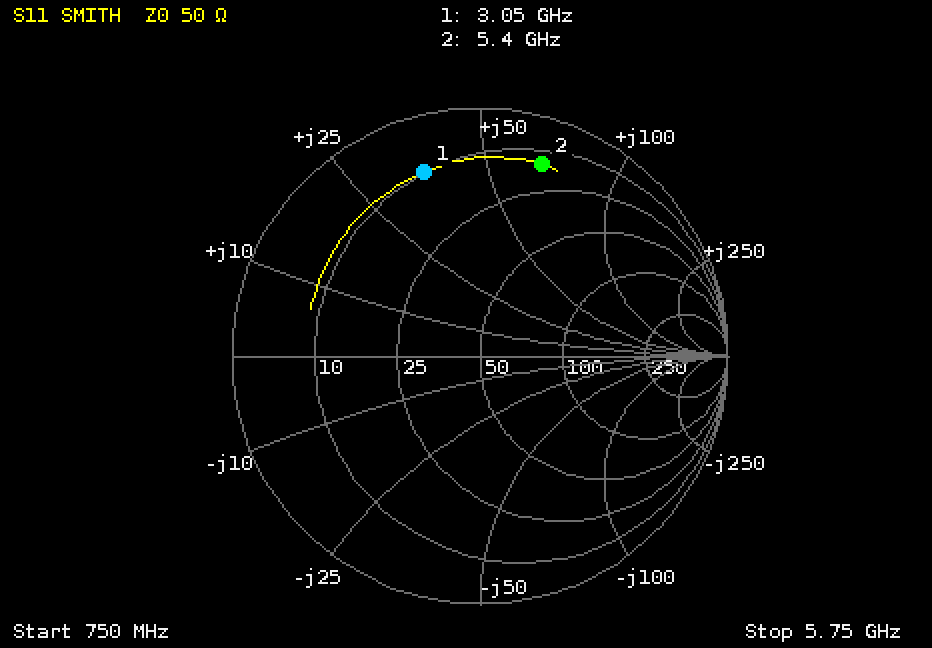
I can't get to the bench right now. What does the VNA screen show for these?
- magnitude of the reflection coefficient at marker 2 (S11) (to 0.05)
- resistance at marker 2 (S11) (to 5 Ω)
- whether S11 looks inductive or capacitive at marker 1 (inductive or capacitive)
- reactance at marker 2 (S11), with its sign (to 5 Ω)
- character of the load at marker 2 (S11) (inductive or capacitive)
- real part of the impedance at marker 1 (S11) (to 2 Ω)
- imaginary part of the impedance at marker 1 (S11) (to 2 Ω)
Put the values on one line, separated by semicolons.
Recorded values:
0.80; 15 Ω; inductive; +65 Ω; inductive; 10 Ω; +36 Ω
